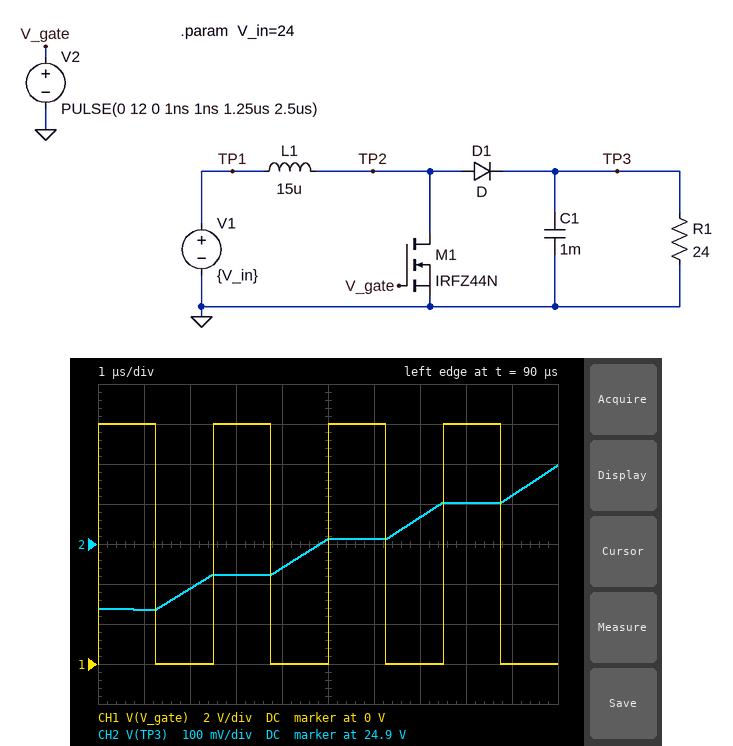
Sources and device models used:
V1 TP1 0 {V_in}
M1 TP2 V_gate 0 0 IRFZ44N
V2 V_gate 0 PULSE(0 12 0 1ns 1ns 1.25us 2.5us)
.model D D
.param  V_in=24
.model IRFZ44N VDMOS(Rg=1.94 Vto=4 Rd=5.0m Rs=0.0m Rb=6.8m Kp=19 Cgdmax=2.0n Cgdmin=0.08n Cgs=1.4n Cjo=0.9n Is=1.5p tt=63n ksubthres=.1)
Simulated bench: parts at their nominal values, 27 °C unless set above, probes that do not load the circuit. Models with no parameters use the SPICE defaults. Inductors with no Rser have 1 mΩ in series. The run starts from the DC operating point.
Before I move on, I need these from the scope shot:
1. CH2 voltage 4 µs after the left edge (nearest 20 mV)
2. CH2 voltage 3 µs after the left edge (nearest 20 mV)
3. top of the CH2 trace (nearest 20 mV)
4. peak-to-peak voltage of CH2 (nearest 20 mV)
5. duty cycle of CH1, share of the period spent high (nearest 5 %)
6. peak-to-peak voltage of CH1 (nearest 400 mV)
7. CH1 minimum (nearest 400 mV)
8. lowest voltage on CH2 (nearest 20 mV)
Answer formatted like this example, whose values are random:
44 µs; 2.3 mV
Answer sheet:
24.84 V; 24.82 V; 25.10 V; 360 mV; 50 %; 12.0 V; 0 V; 24.74 V
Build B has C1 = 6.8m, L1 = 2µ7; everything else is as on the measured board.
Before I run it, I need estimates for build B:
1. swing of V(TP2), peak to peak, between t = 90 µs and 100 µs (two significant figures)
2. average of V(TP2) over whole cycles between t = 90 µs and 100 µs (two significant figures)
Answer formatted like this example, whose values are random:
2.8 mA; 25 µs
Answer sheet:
21 V; 15 V
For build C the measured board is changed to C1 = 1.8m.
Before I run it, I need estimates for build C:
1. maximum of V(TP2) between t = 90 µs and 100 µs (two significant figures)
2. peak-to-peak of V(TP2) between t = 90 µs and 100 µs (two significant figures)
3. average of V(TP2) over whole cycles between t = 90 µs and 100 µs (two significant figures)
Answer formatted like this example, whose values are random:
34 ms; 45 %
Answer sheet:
25 V; 24 V; 13 V
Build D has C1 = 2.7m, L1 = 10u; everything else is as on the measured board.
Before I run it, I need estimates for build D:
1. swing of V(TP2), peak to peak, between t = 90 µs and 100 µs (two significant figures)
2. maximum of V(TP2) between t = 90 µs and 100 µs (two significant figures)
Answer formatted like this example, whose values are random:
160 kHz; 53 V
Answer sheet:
24 V; 25 V
